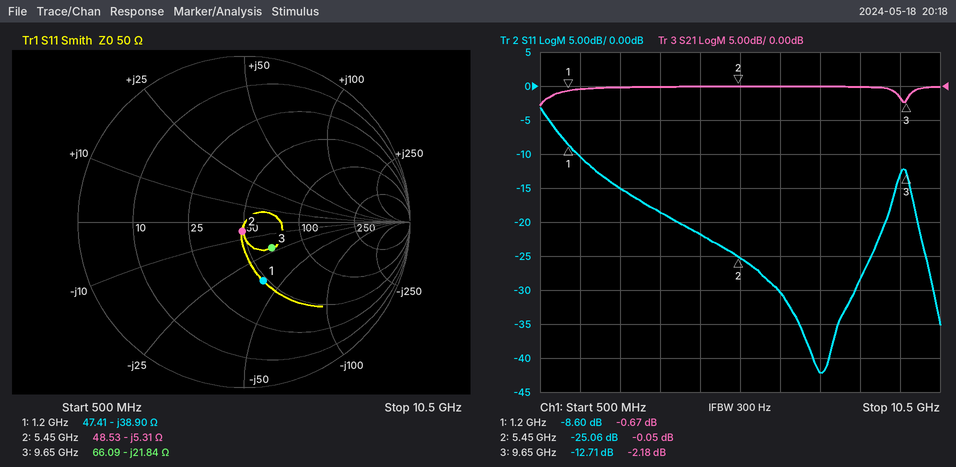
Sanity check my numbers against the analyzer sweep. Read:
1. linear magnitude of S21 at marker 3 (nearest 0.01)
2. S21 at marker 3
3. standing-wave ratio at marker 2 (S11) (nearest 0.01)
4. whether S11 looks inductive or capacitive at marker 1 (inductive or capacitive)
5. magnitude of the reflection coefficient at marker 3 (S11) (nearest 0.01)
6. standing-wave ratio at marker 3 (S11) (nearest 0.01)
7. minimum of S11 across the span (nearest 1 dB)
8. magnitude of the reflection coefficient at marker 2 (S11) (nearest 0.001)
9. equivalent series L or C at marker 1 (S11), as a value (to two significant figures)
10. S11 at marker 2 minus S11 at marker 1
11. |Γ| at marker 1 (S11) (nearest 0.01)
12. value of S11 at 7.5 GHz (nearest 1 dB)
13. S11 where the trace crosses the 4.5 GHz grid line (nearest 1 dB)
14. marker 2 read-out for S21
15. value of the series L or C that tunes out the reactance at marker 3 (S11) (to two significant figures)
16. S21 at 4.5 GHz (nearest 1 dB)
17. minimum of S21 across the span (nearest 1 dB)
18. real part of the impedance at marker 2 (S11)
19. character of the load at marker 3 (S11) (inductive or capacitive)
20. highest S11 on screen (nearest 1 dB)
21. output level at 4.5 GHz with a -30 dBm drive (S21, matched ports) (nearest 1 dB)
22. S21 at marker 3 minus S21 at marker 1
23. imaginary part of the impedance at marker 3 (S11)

0.78
-2.18 dB
1.12
capacitive
0.23
1.60
-42 dB
0.056
3.4 pF
-16.46 dB
0.37
-42 dB
-22 dB
-0.05 dB
360 pH
0 dB
-3 dB
48.53 Ω
capacitive
-3 dB
-30 dBm
-1.51 dB
-21.84 Ω
